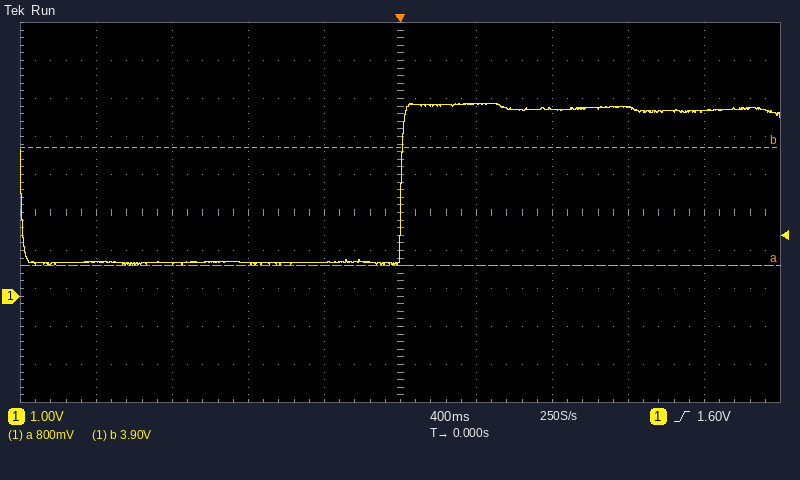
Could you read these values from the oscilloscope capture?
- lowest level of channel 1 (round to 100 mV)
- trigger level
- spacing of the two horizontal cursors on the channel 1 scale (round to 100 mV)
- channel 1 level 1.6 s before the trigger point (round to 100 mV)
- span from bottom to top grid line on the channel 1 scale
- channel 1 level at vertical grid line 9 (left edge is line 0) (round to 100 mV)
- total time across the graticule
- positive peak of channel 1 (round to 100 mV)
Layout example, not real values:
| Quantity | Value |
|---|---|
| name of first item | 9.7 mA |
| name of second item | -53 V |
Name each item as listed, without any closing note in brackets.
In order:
| Quantity | Value |
|---|---|
| lowest level of channel 1 | 800 mV |
| trigger level | 1.60 V |
| spacing of the two horizontal cursors on the channel 1 scale | 3.1 V |
| channel 1 level 1.6 s before the trigger point | 900 mV |
| span from bottom to top grid line on the channel 1 scale | 10 V |
| channel 1 level at vertical grid line 9 (left edge is line 0) | 4.9 V |
| total time across the graticule | 4 s |
| positive peak of channel 1 | 5.1 V |
